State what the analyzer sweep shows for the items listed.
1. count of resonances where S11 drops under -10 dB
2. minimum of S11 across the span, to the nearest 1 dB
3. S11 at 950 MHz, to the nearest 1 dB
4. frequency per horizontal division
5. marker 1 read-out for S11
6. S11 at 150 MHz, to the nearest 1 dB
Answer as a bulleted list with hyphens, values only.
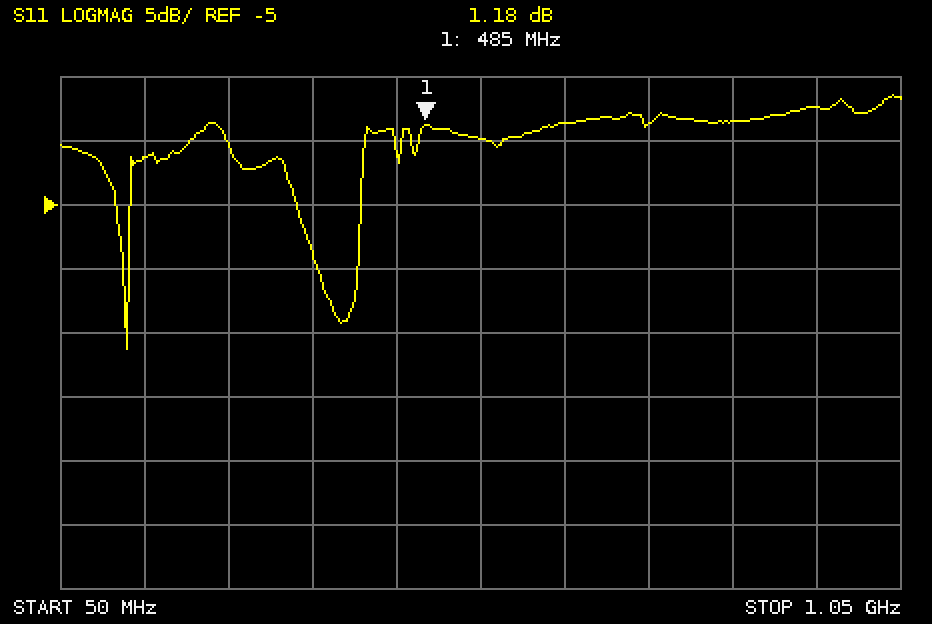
- 2
- -16 dB
- 3 dB
- 100 MHz
- 1.18 dB
- -1 dB
